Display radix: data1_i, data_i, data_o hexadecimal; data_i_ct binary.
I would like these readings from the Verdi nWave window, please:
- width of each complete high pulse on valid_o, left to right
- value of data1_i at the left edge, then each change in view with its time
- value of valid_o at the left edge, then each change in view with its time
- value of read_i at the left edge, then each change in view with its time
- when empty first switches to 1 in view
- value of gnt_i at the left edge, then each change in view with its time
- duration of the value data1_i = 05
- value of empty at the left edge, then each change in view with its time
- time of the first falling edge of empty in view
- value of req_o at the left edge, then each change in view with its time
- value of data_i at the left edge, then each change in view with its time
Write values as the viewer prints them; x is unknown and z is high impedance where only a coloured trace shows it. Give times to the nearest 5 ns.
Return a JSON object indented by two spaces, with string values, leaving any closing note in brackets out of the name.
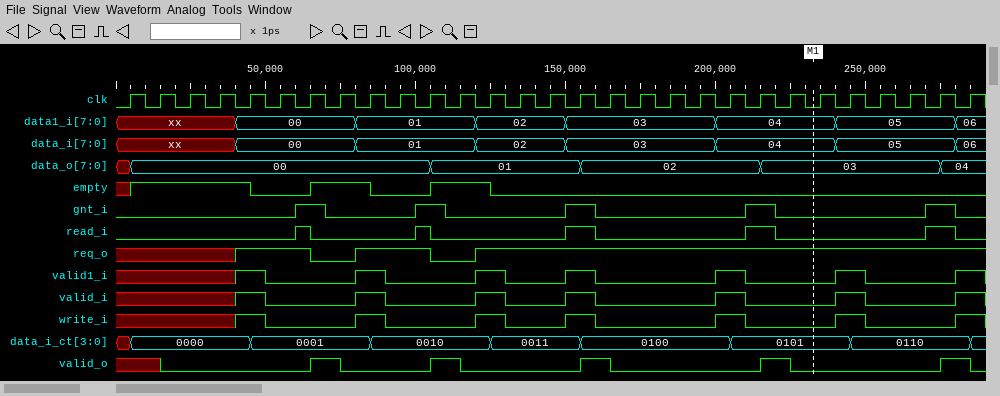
{
  "width of each complete high pulse on valid_o, left to right": "10 ns, 10 ns, 10 ns, 10 ns, 10 ns",
  "value of data1_i at the left edge, then each change in view with its time": "xx, 00 at 40 ns, 01 at 80 ns, 02 at 120 ns, 03 at 150 ns, 04 at 200 ns, 05 at 240 ns, 06 at 280 ns",
  "value of valid_o at the left edge, then each change in view with its time": "x, 0 at 15 ns, 1 at 65 ns, 0 at 75 ns, 1 at 105 ns, 0 at 115 ns, 1 at 155 ns, 0 at 165 ns, 1 at 215 ns, 0 at 225 ns, 1 at 275 ns, 0 at 285 ns",
  "value of read_i at the left edge, then each change in view with its time": "0, 1 at 60 ns, 0 at 65 ns, 1 at 100 ns, 0 at 105 ns, 1 at 150 ns, 0 at 160 ns, 1 at 210 ns, 0 at 220 ns, 1 at 270 ns, 0 at 280 ns",
  "when empty first switches to 1 in view": "5 ns",
  "value of gnt_i at the left edge, then each change in view with its time": "0, 1 at 60 ns, 0 at 70 ns, 1 at 100 ns, 0 at 110 ns, 1 at 150 ns, 0 at 160 ns, 1 at 210 ns, 0 at 220 ns, 1 at 270 ns, 0 at 280 ns",
  "duration of the value data1_i = 05": "40 ns",
  "value of empty at the left edge, then each change in view with its time": "x, 1 at 5 ns, 0 at 45 ns, 1 at 65 ns, 0 at 85 ns, 1 at 105 ns, 0 at 125 ns",
  "time of the first falling edge of empty in view": "45 ns",
  "value of req_o at the left edge, then each change in view with its time": "x, 1 at 40 ns, 0 at 65 ns, 1 at 80 ns, 0 at 105 ns, 1 at 120 ns",
  "value of data_i at the left edge, then each change in view with its time": "xx, 00 at 40 ns, 01 at 80 ns, 02 at 120 ns, 03 at 150 ns, 04 at 200 ns, 05 at 240 ns, 06 at 280 ns"
}
